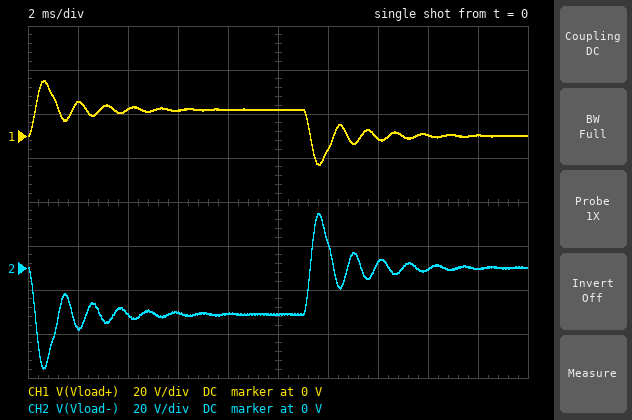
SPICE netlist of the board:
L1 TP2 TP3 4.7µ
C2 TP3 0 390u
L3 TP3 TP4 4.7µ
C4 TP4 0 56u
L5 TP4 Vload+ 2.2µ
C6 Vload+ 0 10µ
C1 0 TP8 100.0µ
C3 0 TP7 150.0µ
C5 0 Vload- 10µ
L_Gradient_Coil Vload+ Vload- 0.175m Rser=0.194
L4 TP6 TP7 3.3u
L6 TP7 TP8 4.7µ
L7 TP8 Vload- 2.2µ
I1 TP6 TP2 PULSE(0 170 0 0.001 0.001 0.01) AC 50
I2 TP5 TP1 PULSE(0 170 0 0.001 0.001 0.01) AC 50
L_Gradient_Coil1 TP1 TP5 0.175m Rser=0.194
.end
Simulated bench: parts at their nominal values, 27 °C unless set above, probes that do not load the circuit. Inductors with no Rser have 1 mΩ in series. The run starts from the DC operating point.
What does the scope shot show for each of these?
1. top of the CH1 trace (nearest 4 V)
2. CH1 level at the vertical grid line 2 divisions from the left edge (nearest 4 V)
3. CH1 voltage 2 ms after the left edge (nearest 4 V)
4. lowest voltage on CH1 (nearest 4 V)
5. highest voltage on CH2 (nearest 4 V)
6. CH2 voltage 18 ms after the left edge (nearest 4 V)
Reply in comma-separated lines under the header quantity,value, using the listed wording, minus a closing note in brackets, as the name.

quantity,value
top of the CH1 trace,24 V
CH1 level at the vertical grid line 2 divisions from the left edge,12 V
CH1 voltage 2 ms after the left edge,16 V
lowest voltage on CH1,-12 V
highest voltage on CH2,24 V
CH2 voltage 18 ms after the left edge,0 V
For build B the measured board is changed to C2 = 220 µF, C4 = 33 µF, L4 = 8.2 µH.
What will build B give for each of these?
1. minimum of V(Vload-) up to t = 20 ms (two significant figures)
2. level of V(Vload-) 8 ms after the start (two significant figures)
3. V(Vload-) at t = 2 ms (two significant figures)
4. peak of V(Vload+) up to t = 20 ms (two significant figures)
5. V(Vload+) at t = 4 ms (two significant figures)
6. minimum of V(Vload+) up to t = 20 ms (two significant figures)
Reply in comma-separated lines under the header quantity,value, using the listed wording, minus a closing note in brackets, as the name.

quantity,value
minimum of V(Vload-) up to t = 20 ms,-35 V
level of V(Vload-) 8 ms after the start,-17 V
V(Vload-) at t = 2 ms,-20 V
peak of V(Vload+) up to t = 20 ms,34 V
V(Vload+) at t = 4 ms,18 V
minimum of V(Vload+) up to t = 20 ms,-18 V
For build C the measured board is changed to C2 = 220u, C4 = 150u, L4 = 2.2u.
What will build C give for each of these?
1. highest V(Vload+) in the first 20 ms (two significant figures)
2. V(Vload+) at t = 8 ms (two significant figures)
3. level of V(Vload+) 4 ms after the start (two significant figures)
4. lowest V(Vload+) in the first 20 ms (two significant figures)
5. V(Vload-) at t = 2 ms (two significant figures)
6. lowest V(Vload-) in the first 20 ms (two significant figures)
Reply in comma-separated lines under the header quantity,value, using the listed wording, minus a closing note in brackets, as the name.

quantity,value
highest V(Vload+) in the first 20 ms,28 V
V(Vload+) at t = 8 ms,13 V
level of V(Vload+) 4 ms after the start,14 V
lowest V(Vload+) in the first 20 ms,-15 V
V(Vload-) at t = 2 ms,-25 V
lowest V(Vload-) in the first 20 ms,-42 V
